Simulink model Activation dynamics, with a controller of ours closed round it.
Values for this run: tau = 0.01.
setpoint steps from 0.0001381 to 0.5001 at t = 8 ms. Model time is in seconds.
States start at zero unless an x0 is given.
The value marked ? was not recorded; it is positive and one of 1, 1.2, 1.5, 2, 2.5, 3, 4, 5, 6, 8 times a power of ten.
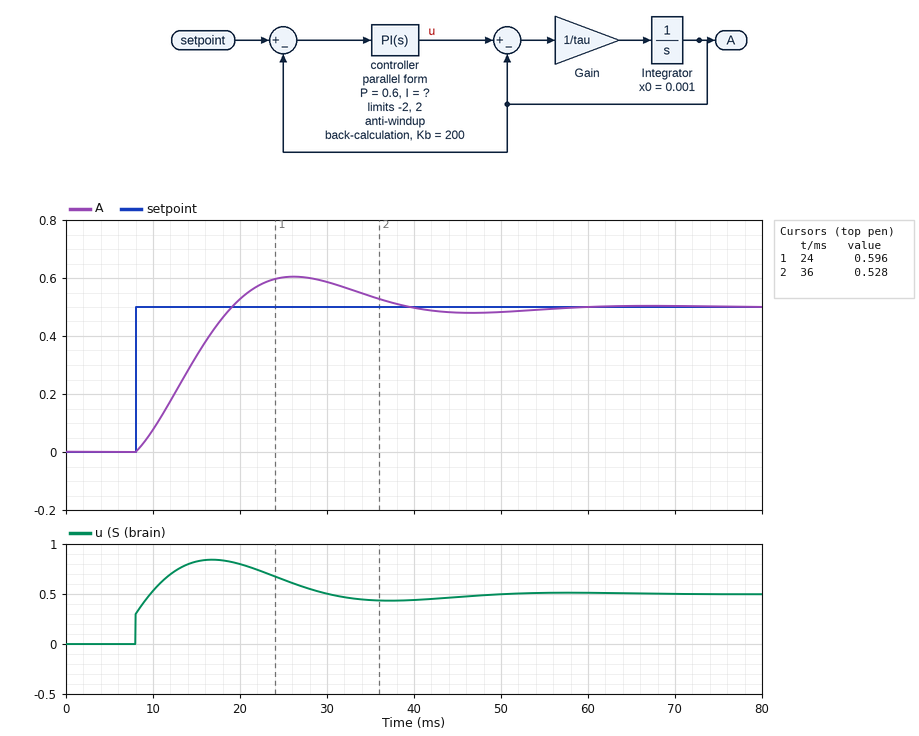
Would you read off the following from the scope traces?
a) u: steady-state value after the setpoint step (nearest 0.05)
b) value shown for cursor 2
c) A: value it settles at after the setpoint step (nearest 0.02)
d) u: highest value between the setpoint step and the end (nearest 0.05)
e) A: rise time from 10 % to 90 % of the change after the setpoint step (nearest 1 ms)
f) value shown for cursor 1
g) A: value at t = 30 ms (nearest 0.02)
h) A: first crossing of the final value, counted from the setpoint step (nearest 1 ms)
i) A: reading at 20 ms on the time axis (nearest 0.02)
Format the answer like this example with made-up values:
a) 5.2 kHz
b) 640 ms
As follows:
a) 0.50
b) 0.528
c) 0.50
d) 0.85
e) 8 ms
f) 0.596
g) 0.58
h) 11 ms
i) 0.52
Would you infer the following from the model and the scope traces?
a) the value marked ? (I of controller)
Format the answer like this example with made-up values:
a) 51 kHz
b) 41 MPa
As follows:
a) 300
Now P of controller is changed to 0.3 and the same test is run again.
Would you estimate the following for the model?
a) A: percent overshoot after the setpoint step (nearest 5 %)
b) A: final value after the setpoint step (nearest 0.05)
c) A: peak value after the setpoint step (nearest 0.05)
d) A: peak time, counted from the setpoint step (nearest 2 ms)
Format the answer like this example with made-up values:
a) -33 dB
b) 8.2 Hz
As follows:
a) 30 %
b) 0.50
c) 0.65
d) 18 ms
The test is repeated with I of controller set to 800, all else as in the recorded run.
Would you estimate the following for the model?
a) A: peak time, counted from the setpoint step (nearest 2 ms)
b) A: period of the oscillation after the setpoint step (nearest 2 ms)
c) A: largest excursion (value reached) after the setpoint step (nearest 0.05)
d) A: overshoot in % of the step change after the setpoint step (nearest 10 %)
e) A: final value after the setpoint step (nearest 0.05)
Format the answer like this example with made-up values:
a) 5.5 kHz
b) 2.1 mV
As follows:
a) 10 ms
b) 24 ms
c) 0.70
d) 40 %
e) 0.50
